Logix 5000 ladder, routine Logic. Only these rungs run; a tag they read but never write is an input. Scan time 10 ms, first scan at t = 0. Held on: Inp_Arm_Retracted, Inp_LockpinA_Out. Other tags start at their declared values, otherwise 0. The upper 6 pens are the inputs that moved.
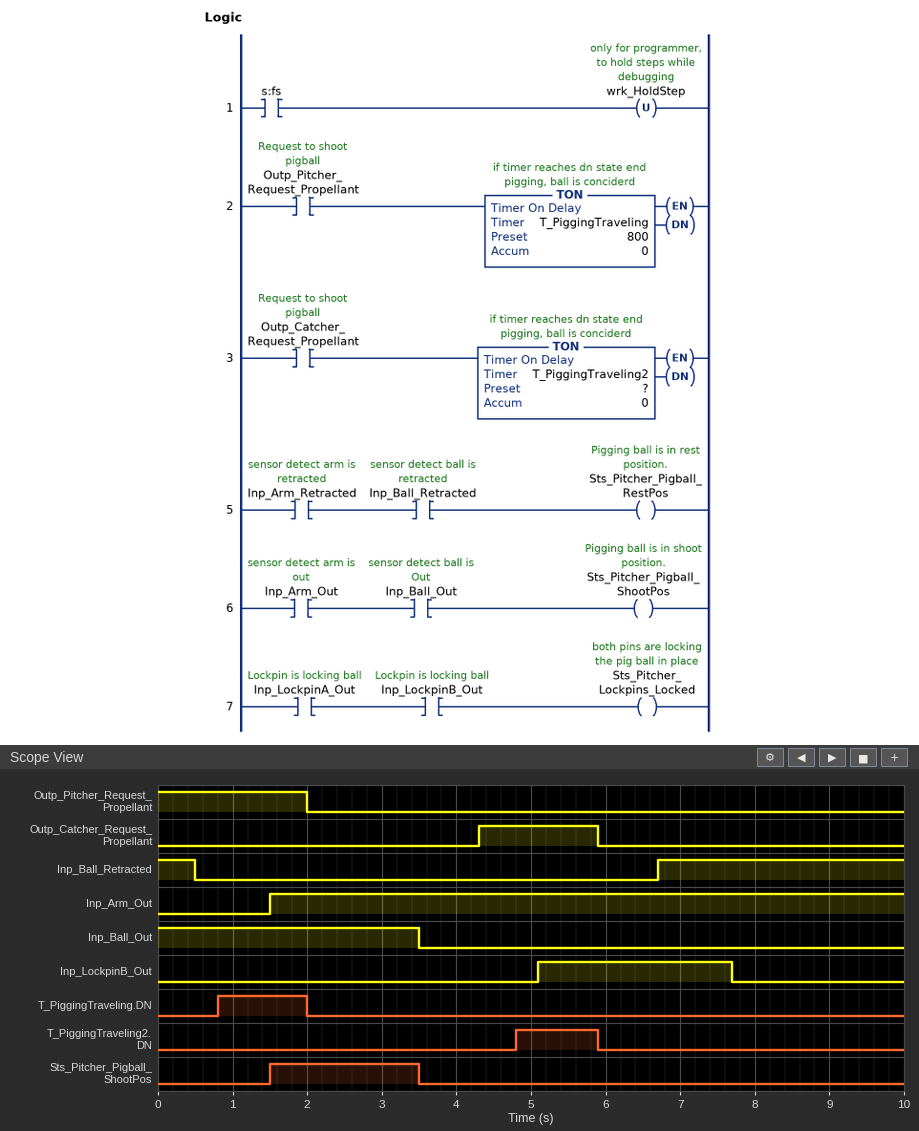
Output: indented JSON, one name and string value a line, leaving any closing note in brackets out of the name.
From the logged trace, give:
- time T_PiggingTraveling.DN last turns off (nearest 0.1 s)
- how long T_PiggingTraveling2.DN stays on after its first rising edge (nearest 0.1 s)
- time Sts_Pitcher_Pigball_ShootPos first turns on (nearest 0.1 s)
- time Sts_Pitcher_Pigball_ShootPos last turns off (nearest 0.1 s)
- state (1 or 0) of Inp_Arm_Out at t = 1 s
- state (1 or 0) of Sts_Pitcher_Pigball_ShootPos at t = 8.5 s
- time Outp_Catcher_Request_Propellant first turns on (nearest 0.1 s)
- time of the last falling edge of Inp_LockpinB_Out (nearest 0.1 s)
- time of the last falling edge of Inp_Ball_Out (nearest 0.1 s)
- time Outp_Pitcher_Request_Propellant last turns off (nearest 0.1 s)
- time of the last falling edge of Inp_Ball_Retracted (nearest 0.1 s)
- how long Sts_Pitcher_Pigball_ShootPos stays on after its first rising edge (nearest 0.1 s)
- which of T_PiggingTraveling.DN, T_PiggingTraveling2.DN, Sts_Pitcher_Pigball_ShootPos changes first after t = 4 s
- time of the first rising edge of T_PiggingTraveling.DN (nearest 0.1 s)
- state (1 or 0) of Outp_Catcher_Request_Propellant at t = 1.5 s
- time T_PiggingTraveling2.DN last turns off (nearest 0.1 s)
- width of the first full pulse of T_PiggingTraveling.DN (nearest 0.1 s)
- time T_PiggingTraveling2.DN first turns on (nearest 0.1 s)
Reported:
{
  "time T_PiggingTraveling.DN last turns off": "2.0 s",
  "how long T_PiggingTraveling2.DN stays on after its first rising edge": "1.1 s",
  "time Sts_Pitcher_Pigball_ShootPos first turns on": "1.5 s",
  "time Sts_Pitcher_Pigball_ShootPos last turns off": "3.5 s",
  "state (1 or 0) of Inp_Arm_Out at t = 1 s": "0",
  "state (1 or 0) of Sts_Pitcher_Pigball_ShootPos at t = 8.5 s": "0",
  "time Outp_Catcher_Request_Propellant first turns on": "4.3 s",
  "time of the last falling edge of Inp_LockpinB_Out": "7.7 s",
  "time of the last falling edge of Inp_Ball_Out": "3.5 s",
  "time Outp_Pitcher_Request_Propellant last turns off": "2.0 s",
  "time of the last falling edge of Inp_Ball_Retracted": "0.5 s",
  "how long Sts_Pitcher_Pigball_ShootPos stays on after its first rising edge": "2.0 s",
  "which of T_PiggingTraveling.DN, T_PiggingTraveling2.DN, Sts_Pitcher_Pigball_ShootPos changes first after t = 4 s": "T_PiggingTraveling2.DN",
  "time of the first rising edge of T_PiggingTraveling.DN": "0.8 s",
  "state (1 or 0) of Outp_Catcher_Request_Propellant at t = 1.5 s": "0",
  "time T_PiggingTraveling2.DN last turns off": "5.9 s",
  "width of the first full pulse of T_PiggingTraveling.DN": "1.2 s",
  "time T_PiggingTraveling2.DN first turns on": "4.8 s"
}
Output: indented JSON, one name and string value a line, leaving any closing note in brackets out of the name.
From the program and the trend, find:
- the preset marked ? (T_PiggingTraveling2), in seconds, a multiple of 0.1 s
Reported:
{
  "the preset marked ? (T_PiggingTraveling2), in seconds, a multiple of 0.1 s": "0.5 s"
}
